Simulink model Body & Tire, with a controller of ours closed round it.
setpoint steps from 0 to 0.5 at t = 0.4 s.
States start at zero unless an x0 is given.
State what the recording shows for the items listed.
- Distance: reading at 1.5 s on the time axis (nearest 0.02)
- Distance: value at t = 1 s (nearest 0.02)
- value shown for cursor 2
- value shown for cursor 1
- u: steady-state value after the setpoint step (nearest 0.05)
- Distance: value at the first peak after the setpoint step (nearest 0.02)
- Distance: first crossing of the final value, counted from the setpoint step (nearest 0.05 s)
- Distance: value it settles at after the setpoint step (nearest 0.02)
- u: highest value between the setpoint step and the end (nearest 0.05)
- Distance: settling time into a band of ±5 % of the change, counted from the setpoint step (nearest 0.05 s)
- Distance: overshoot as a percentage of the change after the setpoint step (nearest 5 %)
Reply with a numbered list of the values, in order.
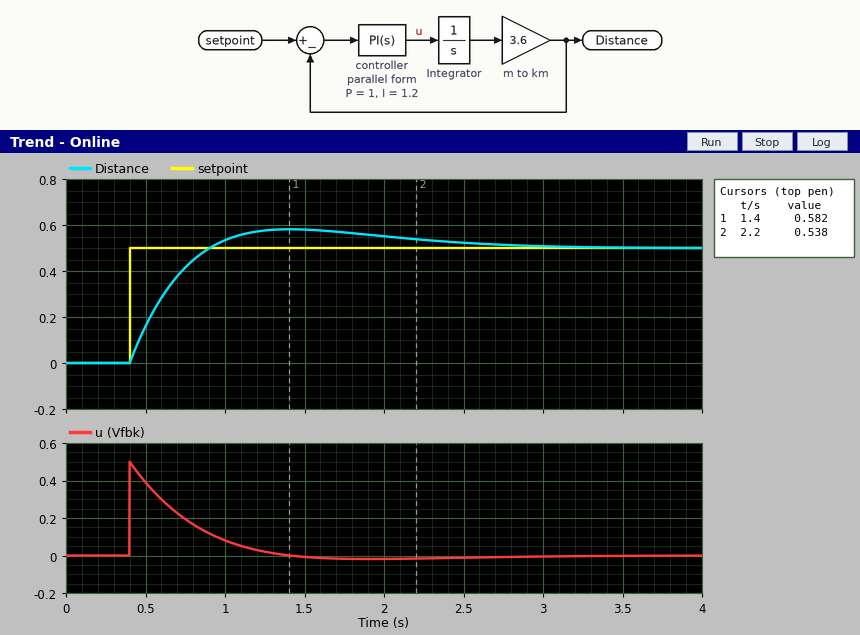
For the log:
1. 0.58
2. 0.54
3. 0.538
4. 0.582
5. 0.00
6. 0.58
7. 0.50 s
8. 0.50
9. 0.50
10. 2.05 s
11. 15 %
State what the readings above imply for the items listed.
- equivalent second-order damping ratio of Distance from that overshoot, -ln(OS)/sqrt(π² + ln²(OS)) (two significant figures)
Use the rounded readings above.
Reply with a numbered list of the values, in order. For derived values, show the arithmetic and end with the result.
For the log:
1. ln(0.15) = -1.897; 1.897 / sqrt(9.870 + 3.599) = 0.52
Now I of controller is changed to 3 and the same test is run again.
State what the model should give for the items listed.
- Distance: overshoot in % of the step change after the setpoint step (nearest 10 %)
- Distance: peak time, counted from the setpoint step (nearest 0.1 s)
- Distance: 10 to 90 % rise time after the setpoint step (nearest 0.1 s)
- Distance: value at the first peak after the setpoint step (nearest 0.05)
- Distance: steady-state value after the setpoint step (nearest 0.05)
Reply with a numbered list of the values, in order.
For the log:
1. 30 %
2. 0.7 s
3. 0.3 s
4. 0.65
5. 0.50
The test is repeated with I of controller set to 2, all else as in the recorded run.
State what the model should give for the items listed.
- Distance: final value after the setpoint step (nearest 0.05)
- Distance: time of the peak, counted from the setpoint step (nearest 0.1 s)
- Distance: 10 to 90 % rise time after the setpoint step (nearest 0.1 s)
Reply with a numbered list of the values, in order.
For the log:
1. 0.50
2. 0.8 s
3. 0.3 s
